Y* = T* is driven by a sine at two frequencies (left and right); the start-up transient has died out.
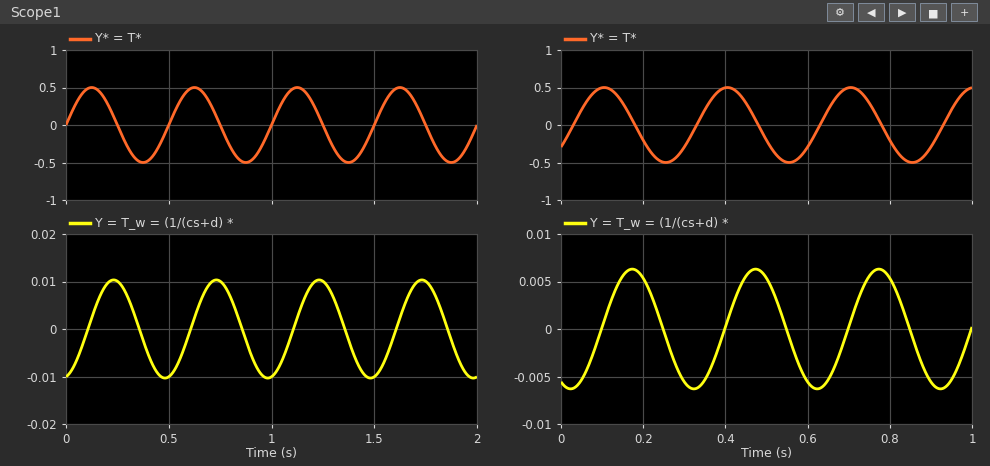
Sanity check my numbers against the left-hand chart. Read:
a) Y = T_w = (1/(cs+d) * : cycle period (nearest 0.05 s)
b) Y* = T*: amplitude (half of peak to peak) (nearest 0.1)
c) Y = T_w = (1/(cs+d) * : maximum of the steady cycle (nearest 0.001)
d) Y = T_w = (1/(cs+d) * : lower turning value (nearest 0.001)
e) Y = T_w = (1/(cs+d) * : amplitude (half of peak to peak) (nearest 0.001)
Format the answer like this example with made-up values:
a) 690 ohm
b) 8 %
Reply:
a) 0.50 s
b) 0.5
c) 0.010
d) -0.010
e) 0.010
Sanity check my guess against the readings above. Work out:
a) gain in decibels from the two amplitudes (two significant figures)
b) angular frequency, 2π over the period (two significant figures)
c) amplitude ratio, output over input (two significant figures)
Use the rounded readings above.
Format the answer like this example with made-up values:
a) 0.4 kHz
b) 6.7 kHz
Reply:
a) -34 dB
b) 13 rad/s
c) 0.020
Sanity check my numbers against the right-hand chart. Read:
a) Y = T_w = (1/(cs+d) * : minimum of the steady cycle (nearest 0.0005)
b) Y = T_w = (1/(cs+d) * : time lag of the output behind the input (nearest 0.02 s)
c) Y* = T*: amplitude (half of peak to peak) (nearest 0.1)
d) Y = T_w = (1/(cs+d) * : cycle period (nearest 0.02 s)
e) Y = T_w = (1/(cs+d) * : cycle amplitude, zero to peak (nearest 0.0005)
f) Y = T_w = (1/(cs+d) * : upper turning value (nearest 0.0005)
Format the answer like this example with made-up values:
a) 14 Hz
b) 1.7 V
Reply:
a) -0.0065
b) 0.06 s
c) 0.5
d) 0.30 s
e) 0.0065
f) 0.0065
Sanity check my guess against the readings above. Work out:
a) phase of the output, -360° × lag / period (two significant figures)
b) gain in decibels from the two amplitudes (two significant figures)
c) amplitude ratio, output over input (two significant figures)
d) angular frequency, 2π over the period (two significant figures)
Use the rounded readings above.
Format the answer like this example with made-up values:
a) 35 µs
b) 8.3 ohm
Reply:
a) -72°
b) -38 dB
c) 0.013
d) 21 rad/s
